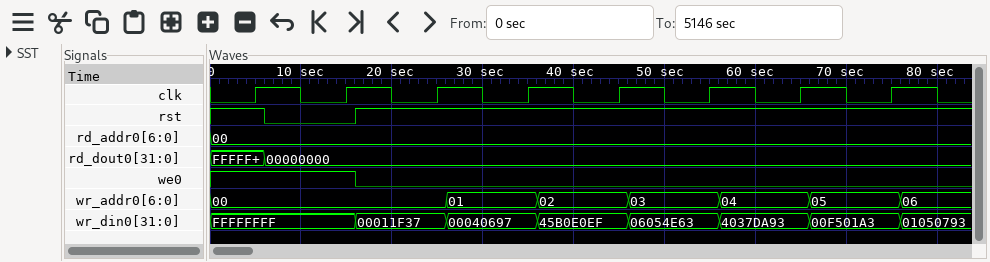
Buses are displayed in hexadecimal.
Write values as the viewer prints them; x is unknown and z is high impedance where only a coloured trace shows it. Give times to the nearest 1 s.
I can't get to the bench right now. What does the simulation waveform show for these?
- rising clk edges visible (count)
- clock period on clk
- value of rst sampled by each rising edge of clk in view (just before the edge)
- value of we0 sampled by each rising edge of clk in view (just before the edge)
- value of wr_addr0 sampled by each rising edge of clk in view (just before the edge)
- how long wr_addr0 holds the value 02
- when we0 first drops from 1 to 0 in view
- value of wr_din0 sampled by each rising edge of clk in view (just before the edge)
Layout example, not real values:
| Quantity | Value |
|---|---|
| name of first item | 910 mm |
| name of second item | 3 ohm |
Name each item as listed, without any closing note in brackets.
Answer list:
| Quantity | Value |
|---|---|
| rising clk edges visible | 8 |
| clock period on clk | 10 s |
| value of rst sampled by each rising edge of clk in view | 1 0 1 1 1 1 1 1 |
| value of we0 sampled by each rising edge of clk in view | 1 1 0 0 0 0 0 0 |
| value of wr_addr0 sampled by each rising edge of clk in view | 00, 00, 00, 01, 02, 03, 04, 05 |
| how long wr_addr0 holds the value 02 | 10 s |
| when we0 first drops from 1 to 0 in view | 16 s |
| value of wr_din0 sampled by each rising edge of clk in view | FFFFFFFF, FFFFFFFF, 00011F37, 00040697, 45B0E0EF, 06054E63, 4037DA93, 00F501A3 |
